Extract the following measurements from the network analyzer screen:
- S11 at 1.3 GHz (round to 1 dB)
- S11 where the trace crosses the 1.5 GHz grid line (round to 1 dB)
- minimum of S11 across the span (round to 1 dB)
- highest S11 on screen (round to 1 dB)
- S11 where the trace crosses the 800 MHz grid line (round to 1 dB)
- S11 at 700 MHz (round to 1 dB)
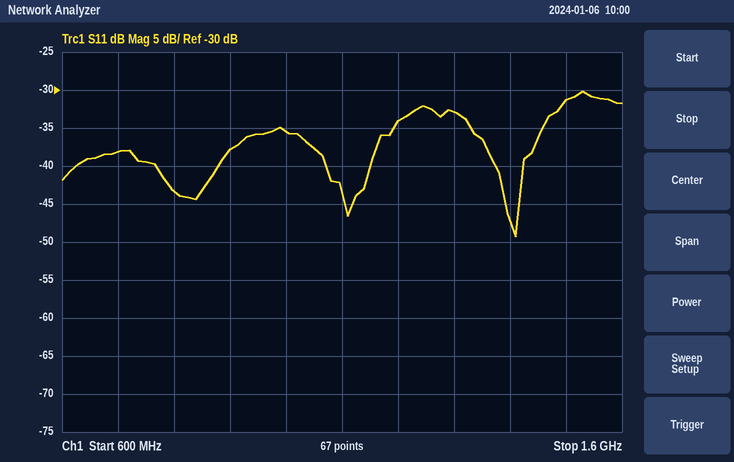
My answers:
-33 dB
-31 dB
-49 dB
-30 dB
-43 dB
-38 dB
